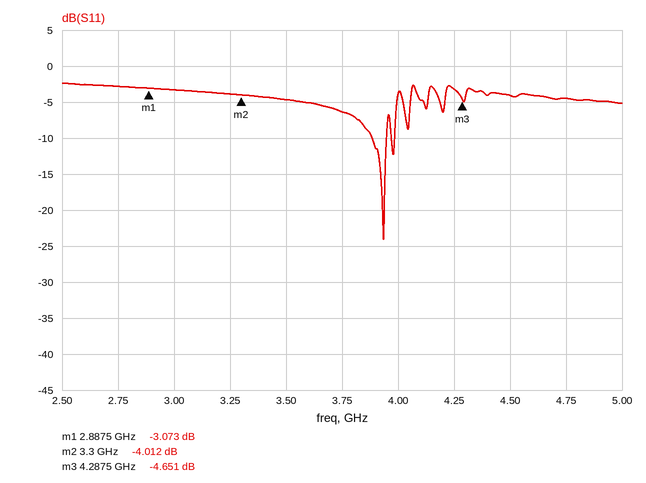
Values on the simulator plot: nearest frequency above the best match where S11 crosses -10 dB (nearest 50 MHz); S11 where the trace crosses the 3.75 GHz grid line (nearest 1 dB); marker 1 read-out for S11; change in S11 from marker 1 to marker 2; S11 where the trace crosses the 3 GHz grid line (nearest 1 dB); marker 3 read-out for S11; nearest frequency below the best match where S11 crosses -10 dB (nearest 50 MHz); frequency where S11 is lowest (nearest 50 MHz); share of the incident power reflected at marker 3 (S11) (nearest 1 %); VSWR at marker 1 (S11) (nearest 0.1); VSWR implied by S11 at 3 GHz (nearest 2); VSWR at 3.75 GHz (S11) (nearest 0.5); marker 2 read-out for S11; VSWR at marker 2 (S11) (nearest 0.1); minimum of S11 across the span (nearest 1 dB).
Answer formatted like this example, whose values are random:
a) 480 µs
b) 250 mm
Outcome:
a) 3.95 GHz
b) -6 dB
c) -3.073 dB
d) -0.939 dB
e) -3 dB
f) -4.651 dB
g) 3.90 GHz
h) 3.95 GHz
i) 34 %
j) 5.7
k) 6
l) 3.0
m) -4.012 dB
n) 4.4
o) -24 dB
